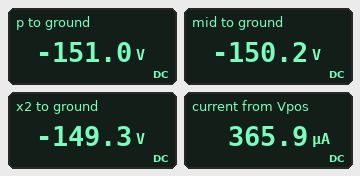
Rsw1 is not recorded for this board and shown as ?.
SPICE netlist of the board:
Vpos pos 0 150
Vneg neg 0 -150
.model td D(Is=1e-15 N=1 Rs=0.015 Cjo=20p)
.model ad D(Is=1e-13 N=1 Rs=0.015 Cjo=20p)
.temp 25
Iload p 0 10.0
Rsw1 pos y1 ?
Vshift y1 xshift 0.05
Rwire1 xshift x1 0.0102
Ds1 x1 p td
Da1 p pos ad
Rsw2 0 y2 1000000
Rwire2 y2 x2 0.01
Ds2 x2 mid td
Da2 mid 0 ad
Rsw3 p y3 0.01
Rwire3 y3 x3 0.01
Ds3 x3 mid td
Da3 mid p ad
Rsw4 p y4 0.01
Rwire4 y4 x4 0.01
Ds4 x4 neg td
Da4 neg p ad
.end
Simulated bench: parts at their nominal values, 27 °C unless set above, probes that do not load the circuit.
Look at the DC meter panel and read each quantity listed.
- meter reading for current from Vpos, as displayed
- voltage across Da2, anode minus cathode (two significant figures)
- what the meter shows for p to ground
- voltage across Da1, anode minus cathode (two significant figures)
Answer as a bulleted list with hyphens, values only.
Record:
- 365.9 µA
- -150 V
- -151.0 V
- -300 V
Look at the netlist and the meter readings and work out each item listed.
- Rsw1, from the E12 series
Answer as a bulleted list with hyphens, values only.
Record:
- 820 kΩ
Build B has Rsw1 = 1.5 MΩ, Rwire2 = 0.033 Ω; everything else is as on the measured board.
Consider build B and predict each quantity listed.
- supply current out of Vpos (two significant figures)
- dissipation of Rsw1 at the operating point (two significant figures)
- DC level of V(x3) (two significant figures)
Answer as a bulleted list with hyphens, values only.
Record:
- 200 µA
- 60 mW
- -150 V
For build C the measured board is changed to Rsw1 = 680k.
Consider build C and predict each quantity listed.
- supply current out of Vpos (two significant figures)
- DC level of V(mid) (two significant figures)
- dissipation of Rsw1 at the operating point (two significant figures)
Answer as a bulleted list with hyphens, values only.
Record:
- 440 µA
- -150 V
- 130 mW
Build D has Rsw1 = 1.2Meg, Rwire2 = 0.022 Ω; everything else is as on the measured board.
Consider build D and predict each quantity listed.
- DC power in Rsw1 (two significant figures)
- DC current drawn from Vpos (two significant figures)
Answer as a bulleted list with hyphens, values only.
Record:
- 75 mW
- 250 µA
